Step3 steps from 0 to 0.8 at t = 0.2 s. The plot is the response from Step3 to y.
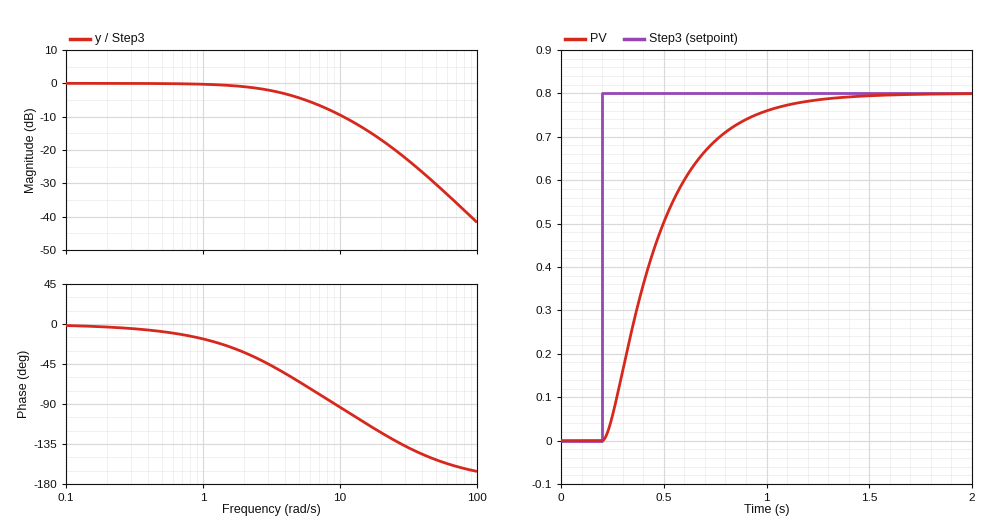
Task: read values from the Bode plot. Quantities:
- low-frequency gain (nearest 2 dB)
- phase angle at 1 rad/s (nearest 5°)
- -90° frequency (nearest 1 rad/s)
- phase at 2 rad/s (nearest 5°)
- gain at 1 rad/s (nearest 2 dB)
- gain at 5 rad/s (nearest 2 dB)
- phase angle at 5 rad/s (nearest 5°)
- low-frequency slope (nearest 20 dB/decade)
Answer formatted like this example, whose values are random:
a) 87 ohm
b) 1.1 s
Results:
a) 0 dB
b) -15°
c) 9 rad/s
d) -30°
e) 0 dB
f) -4 dB
g) -65°
h) 0 dB/decade
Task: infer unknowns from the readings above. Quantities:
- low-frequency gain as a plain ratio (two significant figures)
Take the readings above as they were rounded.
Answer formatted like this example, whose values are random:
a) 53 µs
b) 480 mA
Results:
a) 1.0
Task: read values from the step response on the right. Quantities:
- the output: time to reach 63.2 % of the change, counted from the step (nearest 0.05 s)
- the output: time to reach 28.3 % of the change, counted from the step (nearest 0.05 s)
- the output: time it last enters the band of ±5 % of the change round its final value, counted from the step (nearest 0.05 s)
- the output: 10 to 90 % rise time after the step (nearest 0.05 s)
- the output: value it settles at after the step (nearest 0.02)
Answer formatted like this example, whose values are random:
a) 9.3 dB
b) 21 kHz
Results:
a) 0.30 s
b) 0.15 s
c) 0.80 s
d) 0.55 s
e) 0.80
